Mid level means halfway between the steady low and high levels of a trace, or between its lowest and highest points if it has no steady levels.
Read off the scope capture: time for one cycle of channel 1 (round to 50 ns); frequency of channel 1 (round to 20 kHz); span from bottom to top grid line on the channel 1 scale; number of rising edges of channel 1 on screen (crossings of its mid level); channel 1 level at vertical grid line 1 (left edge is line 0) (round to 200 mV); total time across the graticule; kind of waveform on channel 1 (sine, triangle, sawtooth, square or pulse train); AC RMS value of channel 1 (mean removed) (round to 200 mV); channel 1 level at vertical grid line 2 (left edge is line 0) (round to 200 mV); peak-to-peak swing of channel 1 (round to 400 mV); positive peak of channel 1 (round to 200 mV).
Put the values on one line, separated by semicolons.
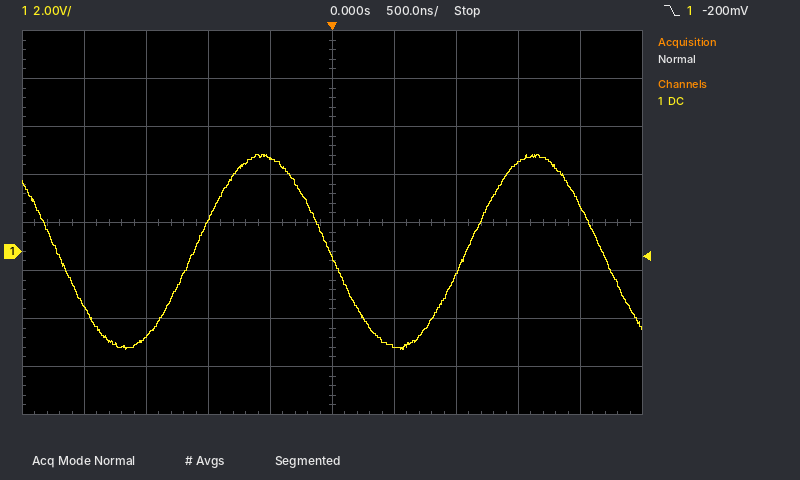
2.20 µs; 460 kHz; 16 V; 2; -2.2 V; 5 µs; sine; 2.8 V; -3.6 V; 8.0 V; 4.0 V
